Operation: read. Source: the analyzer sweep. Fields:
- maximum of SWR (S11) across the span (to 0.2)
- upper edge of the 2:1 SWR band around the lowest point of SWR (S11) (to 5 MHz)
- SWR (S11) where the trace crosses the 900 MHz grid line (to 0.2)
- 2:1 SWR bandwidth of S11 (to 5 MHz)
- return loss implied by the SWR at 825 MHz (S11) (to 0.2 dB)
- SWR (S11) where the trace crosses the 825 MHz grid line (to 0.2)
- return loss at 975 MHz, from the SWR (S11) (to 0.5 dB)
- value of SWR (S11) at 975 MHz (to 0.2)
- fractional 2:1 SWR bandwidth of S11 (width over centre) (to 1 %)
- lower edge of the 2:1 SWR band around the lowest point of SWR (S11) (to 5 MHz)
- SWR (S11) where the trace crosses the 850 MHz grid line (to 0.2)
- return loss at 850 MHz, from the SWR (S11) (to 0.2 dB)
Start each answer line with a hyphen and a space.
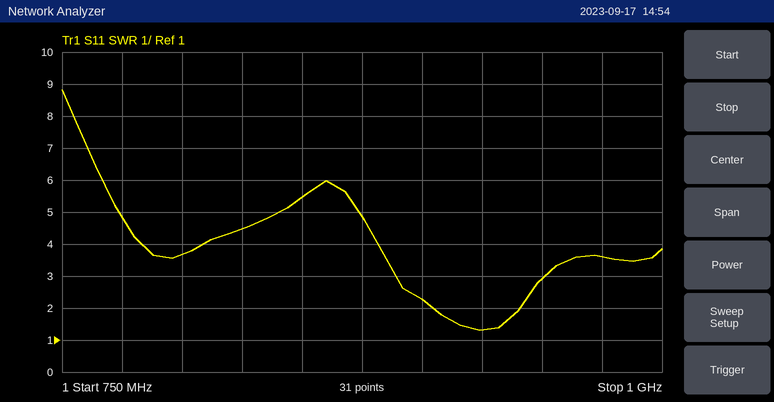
- 8.8
- 940 MHz
- 2.2
- 35 MHz
- 4.0 dB
- 4.4
- 5.0 dB
- 3.6
- 4 %
- 905 MHz
- 5.4
- 3.2 dB
